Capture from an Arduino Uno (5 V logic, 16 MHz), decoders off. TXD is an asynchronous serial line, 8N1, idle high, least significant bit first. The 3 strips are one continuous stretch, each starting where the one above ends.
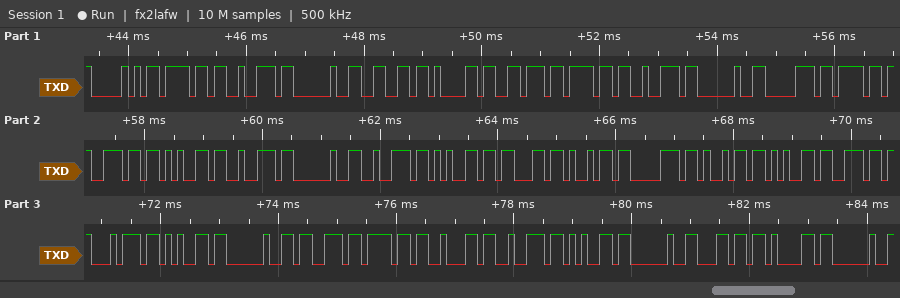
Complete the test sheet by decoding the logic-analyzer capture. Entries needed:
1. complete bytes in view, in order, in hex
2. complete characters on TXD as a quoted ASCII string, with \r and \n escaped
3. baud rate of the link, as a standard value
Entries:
50 6F 72 20 66 61 76 6F 72 20 70 6F 6E 65 72 20 72 65 63 69 70 69 65 6E 74 65 20 73 6F 62 72 65 20 6C 61 20
"Por favor poner recipiente sobre la "
9600 baud
